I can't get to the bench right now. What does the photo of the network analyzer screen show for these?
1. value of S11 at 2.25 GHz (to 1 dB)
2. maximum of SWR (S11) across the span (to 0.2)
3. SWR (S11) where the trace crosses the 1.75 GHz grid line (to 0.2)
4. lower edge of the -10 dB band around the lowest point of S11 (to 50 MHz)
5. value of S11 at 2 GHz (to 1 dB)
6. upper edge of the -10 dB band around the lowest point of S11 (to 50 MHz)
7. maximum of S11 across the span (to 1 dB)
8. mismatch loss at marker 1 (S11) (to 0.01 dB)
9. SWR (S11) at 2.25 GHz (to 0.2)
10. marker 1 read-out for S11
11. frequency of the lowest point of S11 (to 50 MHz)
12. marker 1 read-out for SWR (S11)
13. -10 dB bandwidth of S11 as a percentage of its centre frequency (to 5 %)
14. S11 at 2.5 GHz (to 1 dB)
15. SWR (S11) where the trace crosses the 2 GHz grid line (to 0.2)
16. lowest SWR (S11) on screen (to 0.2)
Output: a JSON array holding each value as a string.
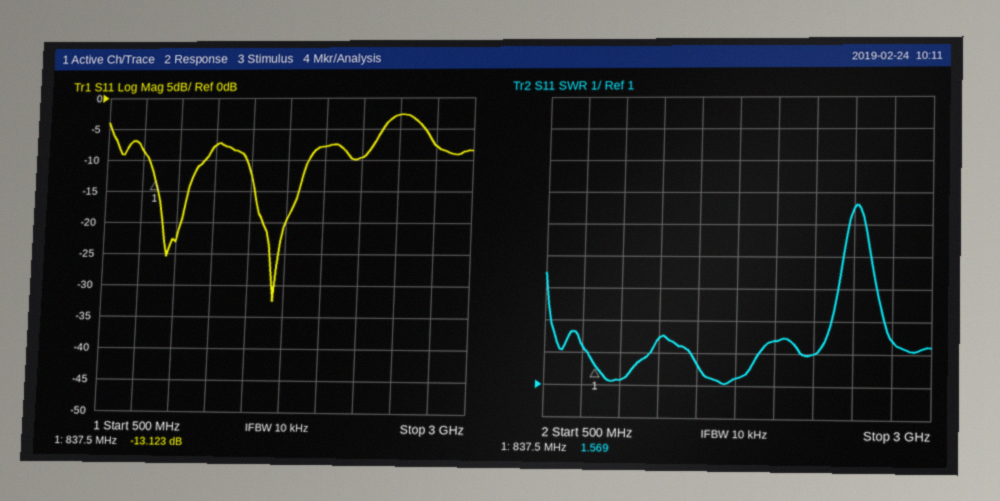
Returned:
["-10 dB", "6.6", "1.2", "1.45 GHz", "-8 dB", "1.90 GHz", "-3 dB", "0.22 dB", "2.0", "-13.123 dB", "1.70 GHz", "1.569", "25 %", "-3 dB", "2.4", "1.0"]
